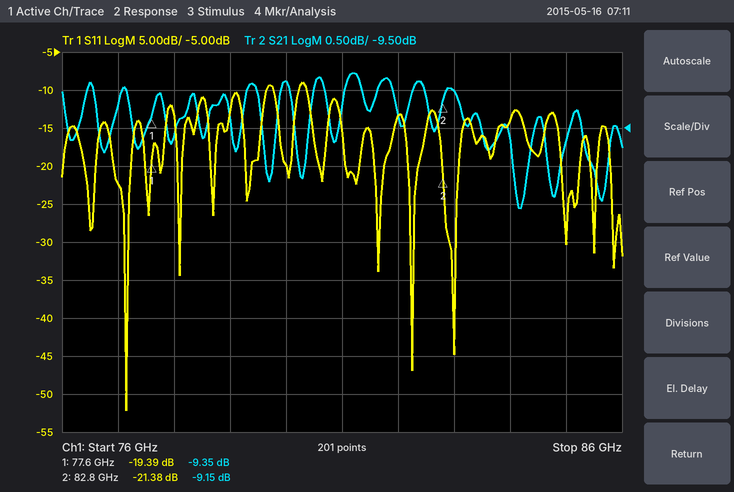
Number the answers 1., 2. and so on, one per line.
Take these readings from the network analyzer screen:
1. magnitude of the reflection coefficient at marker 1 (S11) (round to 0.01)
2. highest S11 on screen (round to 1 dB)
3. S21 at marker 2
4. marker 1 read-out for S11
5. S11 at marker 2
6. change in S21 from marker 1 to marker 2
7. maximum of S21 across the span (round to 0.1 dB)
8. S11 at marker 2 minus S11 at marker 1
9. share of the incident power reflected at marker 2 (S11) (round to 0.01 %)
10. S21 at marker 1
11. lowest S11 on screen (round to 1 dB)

1. 0.11
2. -9 dB
3. -9.15 dB
4. -19.39 dB
5. -21.38 dB
6. 0.20 dB
7. -8.8 dB
8. -1.99 dB
9. 0.73 %
10. -9.35 dB
11. -52 dB
